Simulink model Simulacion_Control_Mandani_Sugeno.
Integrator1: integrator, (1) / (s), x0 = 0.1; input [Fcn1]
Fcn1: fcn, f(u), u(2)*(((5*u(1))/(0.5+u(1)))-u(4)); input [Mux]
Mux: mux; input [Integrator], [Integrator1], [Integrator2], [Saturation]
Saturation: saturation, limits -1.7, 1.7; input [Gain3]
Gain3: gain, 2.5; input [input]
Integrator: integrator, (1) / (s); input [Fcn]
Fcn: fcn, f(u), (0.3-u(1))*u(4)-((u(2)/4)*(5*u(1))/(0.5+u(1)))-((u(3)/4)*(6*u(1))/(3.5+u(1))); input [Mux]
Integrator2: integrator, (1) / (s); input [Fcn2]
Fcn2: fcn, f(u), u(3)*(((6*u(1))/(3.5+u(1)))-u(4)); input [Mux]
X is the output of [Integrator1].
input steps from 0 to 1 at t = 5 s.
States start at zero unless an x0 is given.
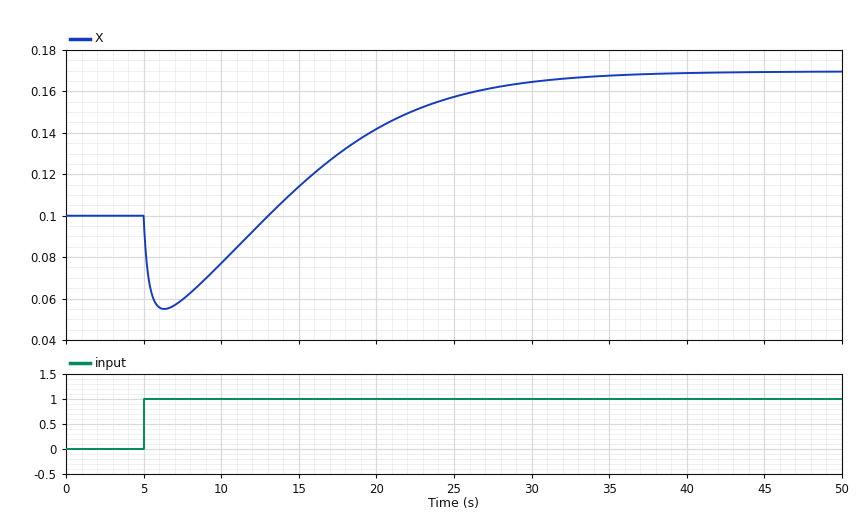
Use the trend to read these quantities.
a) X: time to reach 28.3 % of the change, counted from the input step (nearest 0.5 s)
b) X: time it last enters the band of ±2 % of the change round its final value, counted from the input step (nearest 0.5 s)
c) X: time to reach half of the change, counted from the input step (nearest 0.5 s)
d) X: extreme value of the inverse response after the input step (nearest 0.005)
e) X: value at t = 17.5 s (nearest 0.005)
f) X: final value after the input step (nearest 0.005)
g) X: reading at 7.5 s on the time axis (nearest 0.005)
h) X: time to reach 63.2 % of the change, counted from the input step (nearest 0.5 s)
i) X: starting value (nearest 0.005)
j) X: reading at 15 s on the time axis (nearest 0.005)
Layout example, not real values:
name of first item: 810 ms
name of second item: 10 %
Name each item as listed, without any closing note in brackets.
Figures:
X: time to reach 28.3 % of the change, counted from the input step: 11.0 s
X: time it last enters the band of ±2 % of the change round its final value, counted from the input step: 32.0 s
X: time to reach half of the change, counted from the input step: 13.5 s
X: extreme value of the inverse response after the input step: 0.055
X: value at t = 17.5 s: 0.130
X: final value after the input step: 0.170
X: reading at 7.5 s on the time axis: 0.060
X: time to reach 63.2 % of the change, counted from the input step: 15.5 s
X: starting value: 0.100
X: reading at 15 s on the time axis: 0.115
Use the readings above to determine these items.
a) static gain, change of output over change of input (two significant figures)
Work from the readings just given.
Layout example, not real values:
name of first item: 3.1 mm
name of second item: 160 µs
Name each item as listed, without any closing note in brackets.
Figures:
static gain, change of output over change of input: 0.070
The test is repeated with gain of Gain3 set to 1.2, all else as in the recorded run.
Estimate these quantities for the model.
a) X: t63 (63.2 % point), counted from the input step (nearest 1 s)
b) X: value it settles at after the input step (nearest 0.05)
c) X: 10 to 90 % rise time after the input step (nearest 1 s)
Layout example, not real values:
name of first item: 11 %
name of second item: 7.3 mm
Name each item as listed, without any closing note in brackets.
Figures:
X: t63 (63.2 % point), counted from the input step: 5 s
X: value it settles at after the input step: 0.55
X: 10 to 90 % rise time after the input step: 5 s
